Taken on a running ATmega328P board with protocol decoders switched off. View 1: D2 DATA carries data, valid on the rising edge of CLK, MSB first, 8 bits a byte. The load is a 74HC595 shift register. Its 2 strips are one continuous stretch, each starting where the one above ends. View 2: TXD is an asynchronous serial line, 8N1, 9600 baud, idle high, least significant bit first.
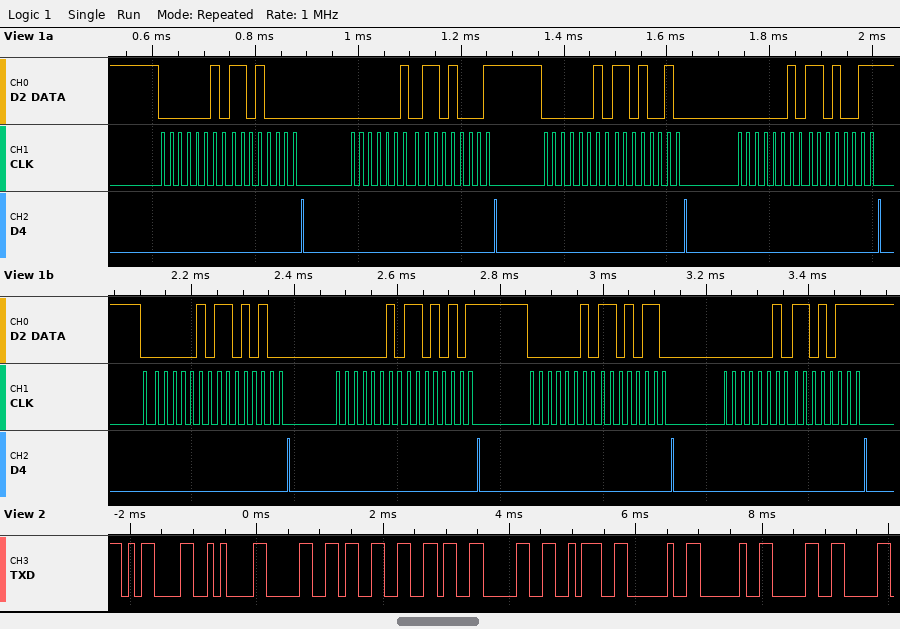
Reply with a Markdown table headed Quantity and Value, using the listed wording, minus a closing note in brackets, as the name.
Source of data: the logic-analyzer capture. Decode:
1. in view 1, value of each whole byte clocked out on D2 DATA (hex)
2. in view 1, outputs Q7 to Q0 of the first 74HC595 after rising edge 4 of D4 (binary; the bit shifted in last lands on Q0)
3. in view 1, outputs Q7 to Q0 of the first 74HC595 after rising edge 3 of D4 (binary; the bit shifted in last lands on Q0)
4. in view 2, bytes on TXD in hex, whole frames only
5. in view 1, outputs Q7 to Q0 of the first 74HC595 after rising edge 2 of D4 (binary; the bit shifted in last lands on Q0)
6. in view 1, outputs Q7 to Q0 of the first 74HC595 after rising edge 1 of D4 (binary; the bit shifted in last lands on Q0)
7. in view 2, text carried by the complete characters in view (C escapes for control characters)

| Quantity | Value |
|---|---|
| in view 1, value of each whole byte clocked out on D2 DATA | 02 D0 02 D1 02 D2 02 D3 02 D4 02 D5 02 D6 02 D7 |
| in view 1, outputs Q7 to Q0 of the first 74HC595 after rising edge 4 of D4 | 11010011 |
| in view 1, outputs Q7 to Q0 of the first 74HC595 after rising edge 3 of D4 | 11010010 |
| in view 2, bytes on TXD in hex, whole frames only | 0x0D 0x0A 0x30 0x33 0x36 0x30 0x3A 0x20 0x20 0x30 |
| in view 1, outputs Q7 to Q0 of the first 74HC595 after rising edge 2 of D4 | 11010001 |
| in view 1, outputs Q7 to Q0 of the first 74HC595 after rising edge 1 of D4 | 11010000 |
| in view 2, text carried by the complete characters in view | "\r\n0360:  0" |
